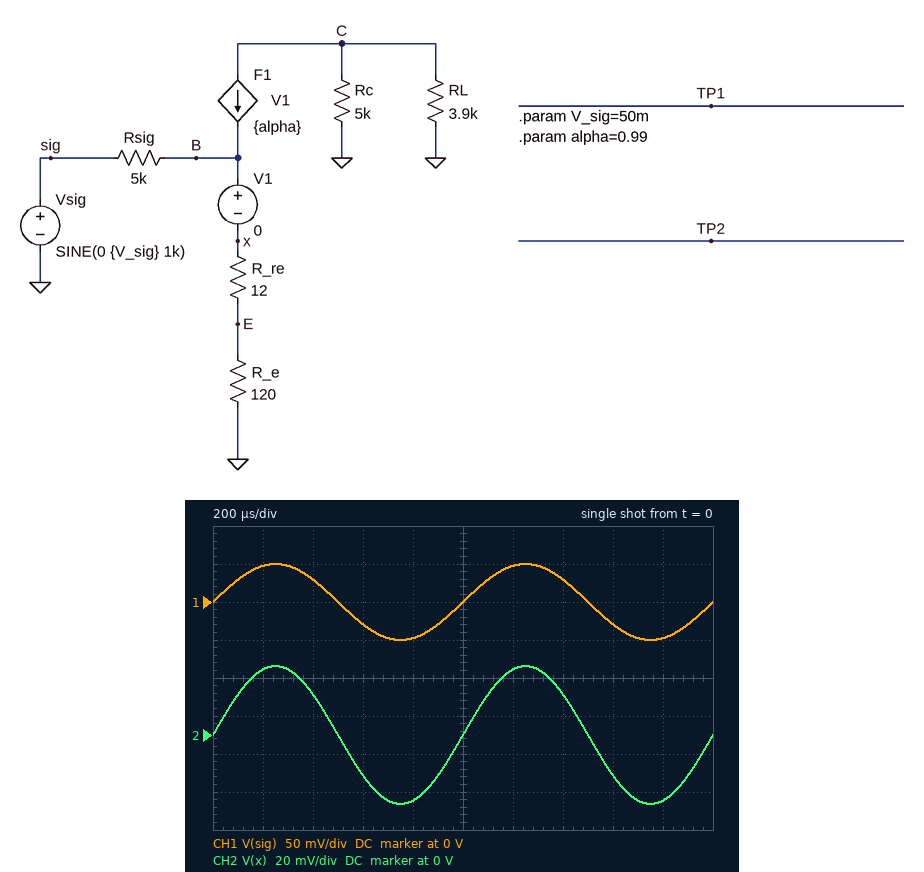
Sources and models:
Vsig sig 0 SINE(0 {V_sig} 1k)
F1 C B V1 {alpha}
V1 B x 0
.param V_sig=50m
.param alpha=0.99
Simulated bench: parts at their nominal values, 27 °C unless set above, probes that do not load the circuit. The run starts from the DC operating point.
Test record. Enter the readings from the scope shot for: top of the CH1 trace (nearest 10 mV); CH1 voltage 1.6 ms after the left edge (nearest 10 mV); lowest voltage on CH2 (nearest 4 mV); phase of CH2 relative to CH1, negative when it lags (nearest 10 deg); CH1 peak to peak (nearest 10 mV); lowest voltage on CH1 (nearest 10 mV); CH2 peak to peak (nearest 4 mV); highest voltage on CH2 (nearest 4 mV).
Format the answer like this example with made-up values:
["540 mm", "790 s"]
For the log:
["50 mV", "-30 mV", "-36 mV", "0 deg", "100 mV", "-50 mV", "72 mV", "36 mV"]
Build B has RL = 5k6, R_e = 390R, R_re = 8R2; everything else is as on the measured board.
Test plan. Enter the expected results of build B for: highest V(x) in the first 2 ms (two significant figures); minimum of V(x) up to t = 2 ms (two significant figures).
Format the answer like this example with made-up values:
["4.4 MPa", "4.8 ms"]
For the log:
["44 mV", "-44 mV"]
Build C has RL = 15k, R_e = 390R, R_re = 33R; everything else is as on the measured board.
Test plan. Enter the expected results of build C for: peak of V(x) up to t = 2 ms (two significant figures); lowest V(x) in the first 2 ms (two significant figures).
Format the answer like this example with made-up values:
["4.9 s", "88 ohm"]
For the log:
["45 mV", "-45 mV"]
